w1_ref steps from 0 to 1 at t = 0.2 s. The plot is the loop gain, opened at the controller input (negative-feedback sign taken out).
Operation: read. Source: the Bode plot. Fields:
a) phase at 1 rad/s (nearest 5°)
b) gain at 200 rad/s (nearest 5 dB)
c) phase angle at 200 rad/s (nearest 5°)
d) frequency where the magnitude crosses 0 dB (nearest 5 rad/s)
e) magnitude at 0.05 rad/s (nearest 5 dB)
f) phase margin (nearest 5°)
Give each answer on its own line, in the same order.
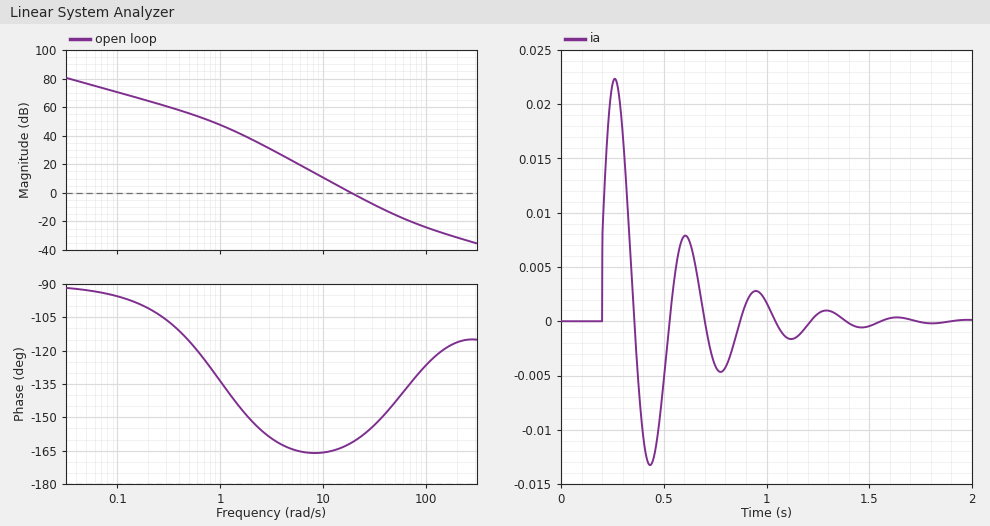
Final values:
-135°
-30 dB
-115°
20 rad/s
75 dB
20°
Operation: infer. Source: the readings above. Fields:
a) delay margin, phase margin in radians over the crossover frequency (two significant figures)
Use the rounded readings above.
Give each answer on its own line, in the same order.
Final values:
0.017 s
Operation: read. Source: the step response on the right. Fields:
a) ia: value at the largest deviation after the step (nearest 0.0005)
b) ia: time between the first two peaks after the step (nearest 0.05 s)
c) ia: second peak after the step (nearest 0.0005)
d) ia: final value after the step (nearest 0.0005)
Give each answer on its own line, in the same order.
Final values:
0.0225
0.35 s
0.0080
0.0000
